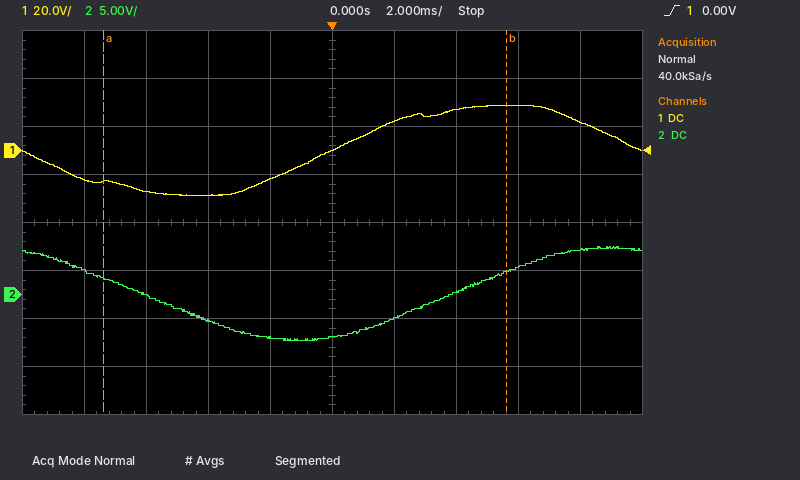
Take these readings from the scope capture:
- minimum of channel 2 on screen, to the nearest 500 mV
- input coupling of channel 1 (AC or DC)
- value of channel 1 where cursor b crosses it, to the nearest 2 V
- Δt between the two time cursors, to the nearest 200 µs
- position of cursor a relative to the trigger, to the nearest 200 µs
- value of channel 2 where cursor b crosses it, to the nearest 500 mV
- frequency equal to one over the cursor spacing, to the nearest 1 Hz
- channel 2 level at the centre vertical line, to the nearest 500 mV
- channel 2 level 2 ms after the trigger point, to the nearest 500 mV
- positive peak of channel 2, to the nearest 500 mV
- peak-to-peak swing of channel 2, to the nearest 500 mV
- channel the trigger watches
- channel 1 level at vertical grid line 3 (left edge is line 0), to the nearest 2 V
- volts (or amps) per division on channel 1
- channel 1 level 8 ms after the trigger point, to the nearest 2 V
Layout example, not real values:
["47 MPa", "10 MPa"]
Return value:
["-5.0 V", "DC", "18 V", "13.0 ms", "-7.4 ms", "2.5 V", "77 Hz", "-4.5 V", "-2.5 V", "5.0 V", "10.0 V", "channel 1", "-18 V", "20 V", "12 V"]
